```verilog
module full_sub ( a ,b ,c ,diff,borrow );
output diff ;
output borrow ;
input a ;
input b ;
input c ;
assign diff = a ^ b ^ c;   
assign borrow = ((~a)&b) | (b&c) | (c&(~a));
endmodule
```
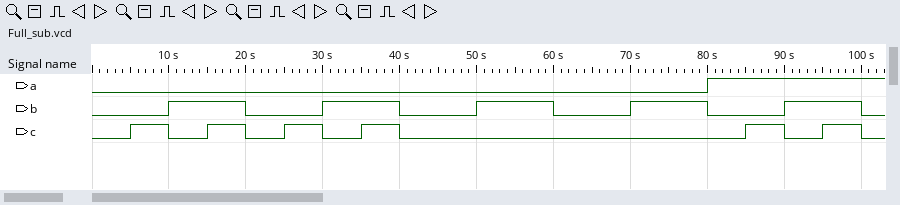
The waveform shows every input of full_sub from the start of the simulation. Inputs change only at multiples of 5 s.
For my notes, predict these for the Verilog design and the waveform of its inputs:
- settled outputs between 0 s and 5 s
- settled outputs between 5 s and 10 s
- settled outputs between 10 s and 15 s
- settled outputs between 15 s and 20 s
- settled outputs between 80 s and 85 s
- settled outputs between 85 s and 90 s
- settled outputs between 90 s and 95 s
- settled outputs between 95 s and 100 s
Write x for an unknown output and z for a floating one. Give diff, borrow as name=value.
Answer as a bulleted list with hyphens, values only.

- diff=0, borrow=0
- diff=1, borrow=1
- diff=1, borrow=1
- diff=0, borrow=1
- diff=1, borrow=0
- diff=0, borrow=0
- diff=0, borrow=0
- diff=1, borrow=1
